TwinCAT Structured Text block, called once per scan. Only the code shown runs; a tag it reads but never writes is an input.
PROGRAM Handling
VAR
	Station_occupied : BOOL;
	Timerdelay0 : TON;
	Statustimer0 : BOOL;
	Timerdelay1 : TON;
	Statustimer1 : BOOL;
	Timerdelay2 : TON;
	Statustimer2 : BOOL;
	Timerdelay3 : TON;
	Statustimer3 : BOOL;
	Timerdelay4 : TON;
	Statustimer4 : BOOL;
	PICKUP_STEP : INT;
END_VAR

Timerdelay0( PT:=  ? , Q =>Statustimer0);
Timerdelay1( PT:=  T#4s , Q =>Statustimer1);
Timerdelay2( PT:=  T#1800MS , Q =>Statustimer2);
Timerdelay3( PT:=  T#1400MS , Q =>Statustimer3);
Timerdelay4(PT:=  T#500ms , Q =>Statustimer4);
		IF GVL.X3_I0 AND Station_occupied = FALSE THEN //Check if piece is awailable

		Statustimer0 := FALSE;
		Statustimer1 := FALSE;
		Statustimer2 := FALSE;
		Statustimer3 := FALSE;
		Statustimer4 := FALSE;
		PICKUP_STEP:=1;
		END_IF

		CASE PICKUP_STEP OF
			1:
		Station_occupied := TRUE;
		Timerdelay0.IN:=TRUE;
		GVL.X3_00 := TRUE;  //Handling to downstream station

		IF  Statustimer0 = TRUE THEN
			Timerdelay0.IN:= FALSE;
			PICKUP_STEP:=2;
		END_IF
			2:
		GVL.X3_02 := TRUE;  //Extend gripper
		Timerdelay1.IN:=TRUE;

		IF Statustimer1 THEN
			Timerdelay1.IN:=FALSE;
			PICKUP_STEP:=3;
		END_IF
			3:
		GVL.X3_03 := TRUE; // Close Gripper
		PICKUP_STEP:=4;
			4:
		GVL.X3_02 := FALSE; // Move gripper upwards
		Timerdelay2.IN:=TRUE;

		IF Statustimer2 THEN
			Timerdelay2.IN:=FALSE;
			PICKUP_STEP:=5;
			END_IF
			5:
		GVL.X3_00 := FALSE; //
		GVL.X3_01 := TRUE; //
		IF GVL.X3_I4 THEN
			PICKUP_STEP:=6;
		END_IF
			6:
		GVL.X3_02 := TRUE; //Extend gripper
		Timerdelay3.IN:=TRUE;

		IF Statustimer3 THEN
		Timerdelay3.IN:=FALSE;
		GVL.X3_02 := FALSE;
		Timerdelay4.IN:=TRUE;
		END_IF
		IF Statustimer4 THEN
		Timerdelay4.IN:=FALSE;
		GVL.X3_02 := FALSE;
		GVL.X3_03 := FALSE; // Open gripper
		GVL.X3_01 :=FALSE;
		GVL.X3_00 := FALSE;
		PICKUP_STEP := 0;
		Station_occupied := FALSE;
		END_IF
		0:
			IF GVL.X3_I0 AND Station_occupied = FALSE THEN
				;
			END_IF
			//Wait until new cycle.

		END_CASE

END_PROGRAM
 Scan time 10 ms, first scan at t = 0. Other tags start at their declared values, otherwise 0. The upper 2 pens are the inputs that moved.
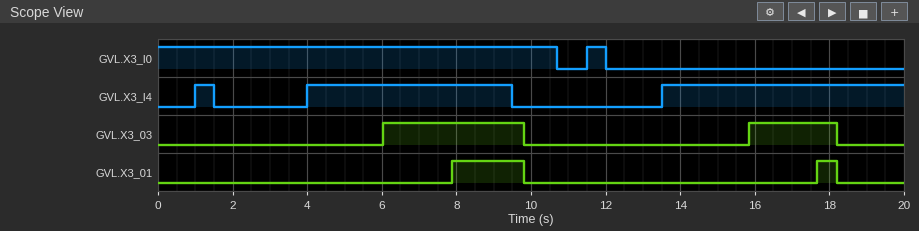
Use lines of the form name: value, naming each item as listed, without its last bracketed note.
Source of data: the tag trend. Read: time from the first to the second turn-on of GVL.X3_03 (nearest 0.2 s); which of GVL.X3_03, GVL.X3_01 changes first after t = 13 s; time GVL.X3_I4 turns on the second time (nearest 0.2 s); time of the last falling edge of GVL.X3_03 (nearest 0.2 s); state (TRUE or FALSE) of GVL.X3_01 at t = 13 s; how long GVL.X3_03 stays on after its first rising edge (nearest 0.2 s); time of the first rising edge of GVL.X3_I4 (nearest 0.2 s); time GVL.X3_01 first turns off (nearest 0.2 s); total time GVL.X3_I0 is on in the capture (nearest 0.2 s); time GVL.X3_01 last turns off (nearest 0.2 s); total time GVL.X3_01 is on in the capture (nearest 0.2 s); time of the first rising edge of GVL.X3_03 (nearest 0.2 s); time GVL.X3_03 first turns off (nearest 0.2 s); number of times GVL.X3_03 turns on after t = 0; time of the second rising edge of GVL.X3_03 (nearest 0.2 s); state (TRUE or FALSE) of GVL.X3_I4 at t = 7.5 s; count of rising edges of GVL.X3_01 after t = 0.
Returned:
time from the first to the second turn-on of GVL.X3_03: 9.8 s
which of GVL.X3_03, GVL.X3_01 changes first after t = 13 s: GVL.X3_03
time GVL.X3_I4 turns on the second time: 4.0 s
time of the last falling edge of GVL.X3_03: 18.2 s
state (TRUE or FALSE) of GVL.X3_01 at t = 13 s: FALSE
how long GVL.X3_03 stays on after its first rising edge: 3.8 s
time of the first rising edge of GVL.X3_I4: 1.0 s
time GVL.X3_01 first turns off: 9.8 s
total time GVL.X3_I0 is on in the capture: 11.2 s
time GVL.X3_01 last turns off: 18.2 s
total time GVL.X3_01 is on in the capture: 2.4 s
time of the first rising edge of GVL.X3_03: 6.0 s
time GVL.X3_03 first turns off: 9.8 s
number of times GVL.X3_03 turns on after t = 0: 2
time of the second rising edge of GVL.X3_03: 15.8 s
state (TRUE or FALSE) of GVL.X3_I4 at t = 7.5 s: TRUE
count of rising edges of GVL.X3_01 after t = 0: 2
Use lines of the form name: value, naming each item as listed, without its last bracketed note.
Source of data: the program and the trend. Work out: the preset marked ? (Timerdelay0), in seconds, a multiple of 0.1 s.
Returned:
the preset marked ? (Timerdelay0), in seconds, a multiple of 0.1 s: 2.0 s
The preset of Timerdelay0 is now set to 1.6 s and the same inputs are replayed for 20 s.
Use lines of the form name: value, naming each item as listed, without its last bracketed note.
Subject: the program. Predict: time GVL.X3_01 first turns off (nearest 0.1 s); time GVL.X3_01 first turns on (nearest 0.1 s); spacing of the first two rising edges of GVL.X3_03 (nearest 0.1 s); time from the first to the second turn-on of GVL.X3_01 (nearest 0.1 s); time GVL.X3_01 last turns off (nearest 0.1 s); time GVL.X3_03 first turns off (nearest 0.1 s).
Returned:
time GVL.X3_01 first turns off: 9.4 s
time GVL.X3_01 first turns on: 7.5 s
spacing of the first two rising edges of GVL.X3_03: 9.4 s
time from the first to the second turn-on of GVL.X3_01: 9.4 s
time GVL.X3_01 last turns off: 17.4 s
time GVL.X3_03 first turns off: 9.4 s
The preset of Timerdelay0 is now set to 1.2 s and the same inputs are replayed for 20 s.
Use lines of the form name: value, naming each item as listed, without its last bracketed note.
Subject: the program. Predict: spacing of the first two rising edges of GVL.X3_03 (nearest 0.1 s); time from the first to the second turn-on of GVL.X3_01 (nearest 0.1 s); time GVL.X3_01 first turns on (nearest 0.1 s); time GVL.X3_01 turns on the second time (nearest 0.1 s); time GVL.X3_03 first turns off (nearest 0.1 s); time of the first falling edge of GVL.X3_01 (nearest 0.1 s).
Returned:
spacing of the first two rising edges of GVL.X3_03: 9.0 s
time from the first to the second turn-on of GVL.X3_01: 9.0 s
time GVL.X3_01 first turns on: 7.1 s
time GVL.X3_01 turns on the second time: 16.1 s
time GVL.X3_03 first turns off: 9.0 s
time of the first falling edge of GVL.X3_01: 9.0 s
